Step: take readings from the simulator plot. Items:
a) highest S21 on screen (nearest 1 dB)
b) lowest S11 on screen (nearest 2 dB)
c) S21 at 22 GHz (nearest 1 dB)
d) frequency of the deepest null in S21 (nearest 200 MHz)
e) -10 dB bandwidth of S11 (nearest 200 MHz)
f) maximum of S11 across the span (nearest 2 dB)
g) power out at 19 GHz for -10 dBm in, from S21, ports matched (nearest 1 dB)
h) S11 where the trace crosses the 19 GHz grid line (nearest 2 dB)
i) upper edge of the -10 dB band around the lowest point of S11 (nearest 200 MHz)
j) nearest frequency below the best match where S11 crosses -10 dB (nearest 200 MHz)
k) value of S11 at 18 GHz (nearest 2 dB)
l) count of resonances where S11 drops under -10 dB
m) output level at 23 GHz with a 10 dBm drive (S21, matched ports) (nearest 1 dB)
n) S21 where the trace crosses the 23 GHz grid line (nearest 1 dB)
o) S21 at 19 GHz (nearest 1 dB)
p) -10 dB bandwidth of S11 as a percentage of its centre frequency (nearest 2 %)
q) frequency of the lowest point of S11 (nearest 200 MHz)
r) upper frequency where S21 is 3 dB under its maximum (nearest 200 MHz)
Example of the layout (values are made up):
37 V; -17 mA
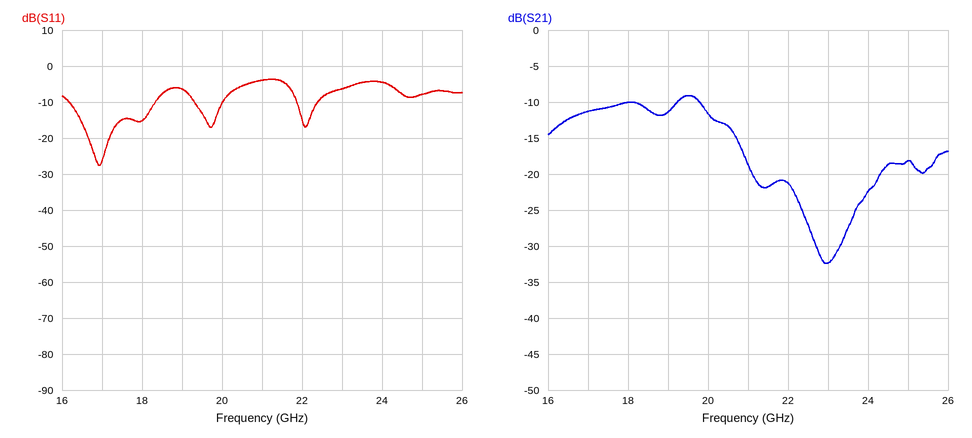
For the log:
-9 dB; -28 dB; -21 dB; 23.0 GHz; 2.2 GHz; -4 dB; -21 dBm; -6 dB; 18.4 GHz; 16.2 GHz; -16 dB; 3; -22 dBm; -32 dB; -11 dB; 12 %; 17.0 GHz; 20.0 GHz
